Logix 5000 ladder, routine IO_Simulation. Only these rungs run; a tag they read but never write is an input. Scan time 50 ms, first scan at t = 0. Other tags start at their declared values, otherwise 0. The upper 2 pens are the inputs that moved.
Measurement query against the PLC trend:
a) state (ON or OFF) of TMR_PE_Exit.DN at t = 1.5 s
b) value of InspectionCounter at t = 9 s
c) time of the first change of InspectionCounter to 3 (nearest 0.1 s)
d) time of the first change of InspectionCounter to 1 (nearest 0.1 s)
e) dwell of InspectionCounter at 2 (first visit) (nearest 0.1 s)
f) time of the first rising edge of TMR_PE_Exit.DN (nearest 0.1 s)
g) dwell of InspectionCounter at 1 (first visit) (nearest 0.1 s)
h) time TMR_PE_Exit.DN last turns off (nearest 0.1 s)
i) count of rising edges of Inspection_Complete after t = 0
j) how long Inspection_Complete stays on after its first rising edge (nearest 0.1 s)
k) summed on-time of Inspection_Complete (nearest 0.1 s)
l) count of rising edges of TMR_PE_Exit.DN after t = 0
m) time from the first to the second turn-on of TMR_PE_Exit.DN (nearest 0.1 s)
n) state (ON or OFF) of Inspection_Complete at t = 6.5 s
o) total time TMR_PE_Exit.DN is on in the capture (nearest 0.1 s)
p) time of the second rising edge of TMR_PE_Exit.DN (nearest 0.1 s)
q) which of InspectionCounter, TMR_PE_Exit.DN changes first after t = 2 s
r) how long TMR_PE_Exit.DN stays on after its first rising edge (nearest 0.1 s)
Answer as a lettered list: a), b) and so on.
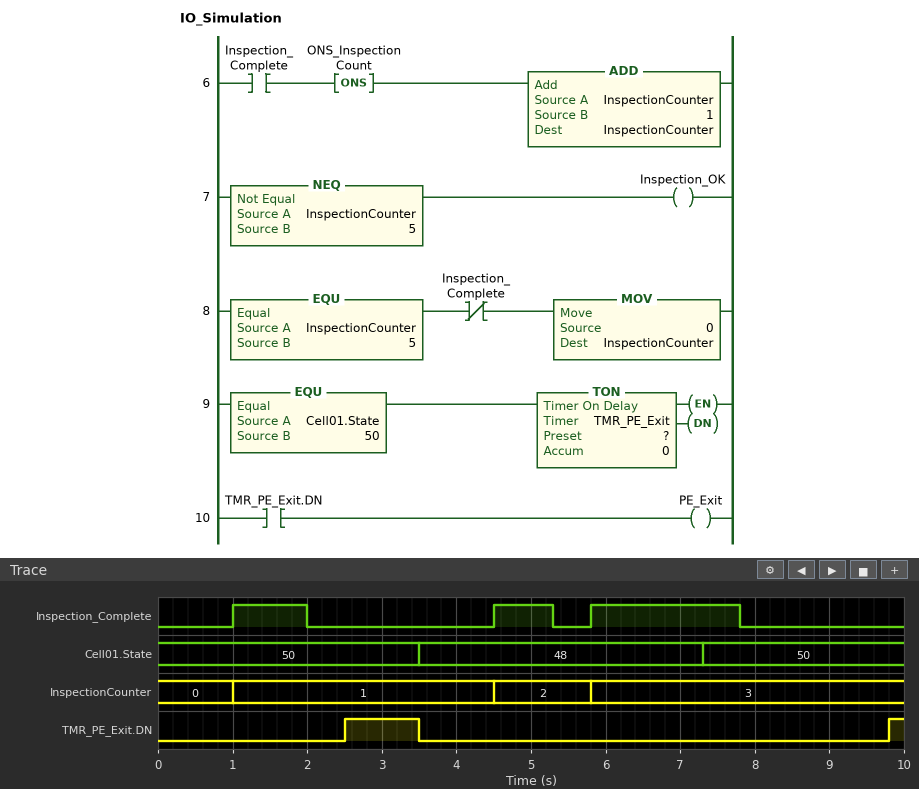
a) OFF
b) 3
c) 5.8 s
d) 1.0 s
e) 1.3 s
f) 2.5 s
g) 3.5 s
h) 3.5 s
i) 3
j) 1.0 s
k) 3.8 s
l) 2
m) 7.3 s
n) ON
o) 1.2 s
p) 9.8 s
q) TMR_PE_Exit.DN
r) 1.0 s
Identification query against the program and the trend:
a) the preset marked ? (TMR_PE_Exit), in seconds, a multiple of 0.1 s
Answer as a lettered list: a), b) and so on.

a) 2.5 s
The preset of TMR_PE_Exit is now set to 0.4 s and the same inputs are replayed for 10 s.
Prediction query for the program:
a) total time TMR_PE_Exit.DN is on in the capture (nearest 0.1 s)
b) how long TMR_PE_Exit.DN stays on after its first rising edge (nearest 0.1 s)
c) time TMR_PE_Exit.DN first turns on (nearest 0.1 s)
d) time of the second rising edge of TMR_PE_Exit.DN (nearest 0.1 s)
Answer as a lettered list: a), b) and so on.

a) 5.4 s
b) 3.1 s
c) 0.4 s
d) 7.7 s
